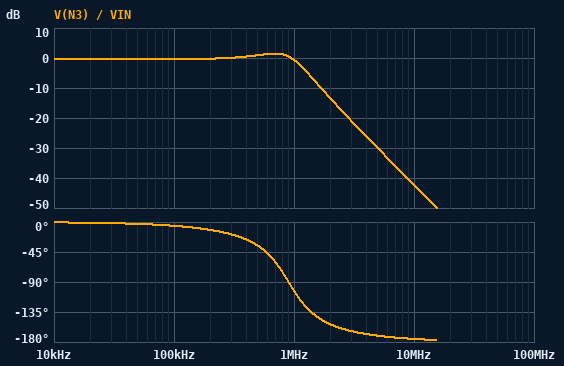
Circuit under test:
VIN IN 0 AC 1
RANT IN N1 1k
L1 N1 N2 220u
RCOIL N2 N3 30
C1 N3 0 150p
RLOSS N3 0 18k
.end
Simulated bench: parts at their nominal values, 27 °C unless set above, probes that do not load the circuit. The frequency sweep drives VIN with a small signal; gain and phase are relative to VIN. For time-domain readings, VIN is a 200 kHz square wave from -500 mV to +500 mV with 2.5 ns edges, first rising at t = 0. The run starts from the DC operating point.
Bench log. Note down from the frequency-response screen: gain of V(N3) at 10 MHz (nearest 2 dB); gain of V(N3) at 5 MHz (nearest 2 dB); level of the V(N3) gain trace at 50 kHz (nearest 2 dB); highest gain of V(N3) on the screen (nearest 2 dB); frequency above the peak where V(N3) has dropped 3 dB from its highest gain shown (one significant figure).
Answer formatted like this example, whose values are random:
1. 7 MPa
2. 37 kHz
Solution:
1. -42 dB
2. -30 dB
3. 0 dB
4. 2 dB
5. 1 MHz
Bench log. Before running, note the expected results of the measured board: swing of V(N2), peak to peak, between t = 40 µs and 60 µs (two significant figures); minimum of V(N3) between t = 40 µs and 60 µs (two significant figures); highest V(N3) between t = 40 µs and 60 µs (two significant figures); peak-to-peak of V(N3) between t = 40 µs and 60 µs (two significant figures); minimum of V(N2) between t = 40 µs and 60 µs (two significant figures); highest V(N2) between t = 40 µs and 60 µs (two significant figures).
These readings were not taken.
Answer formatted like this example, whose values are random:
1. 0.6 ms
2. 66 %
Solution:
1. 1.3 V
2. -670 mV
3. 670 mV
4. 1.3 V
5. -670 mV
6. 670 mV
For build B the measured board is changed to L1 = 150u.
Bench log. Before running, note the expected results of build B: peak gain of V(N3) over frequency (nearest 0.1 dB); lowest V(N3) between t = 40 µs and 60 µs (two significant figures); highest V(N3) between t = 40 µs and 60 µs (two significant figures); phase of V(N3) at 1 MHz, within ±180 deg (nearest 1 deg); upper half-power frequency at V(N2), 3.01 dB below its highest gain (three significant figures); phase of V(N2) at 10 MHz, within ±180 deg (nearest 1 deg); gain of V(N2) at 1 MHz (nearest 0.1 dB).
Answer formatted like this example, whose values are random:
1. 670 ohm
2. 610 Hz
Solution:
1. 0.5 dB
2. -610 mV
3. 610 mV
4. -81 deg
5. 1.26 MHz
6. -158 deg
7. -0.3 dB
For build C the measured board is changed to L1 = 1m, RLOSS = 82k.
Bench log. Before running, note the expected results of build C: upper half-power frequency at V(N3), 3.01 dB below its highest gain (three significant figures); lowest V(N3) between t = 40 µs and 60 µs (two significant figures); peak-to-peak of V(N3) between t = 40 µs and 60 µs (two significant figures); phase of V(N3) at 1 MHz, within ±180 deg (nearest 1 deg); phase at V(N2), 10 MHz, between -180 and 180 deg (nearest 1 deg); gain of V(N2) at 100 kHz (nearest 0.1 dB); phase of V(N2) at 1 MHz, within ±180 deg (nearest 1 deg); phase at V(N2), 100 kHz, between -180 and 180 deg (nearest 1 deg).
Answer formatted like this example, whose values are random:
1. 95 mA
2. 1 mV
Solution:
1. 476 kHz
2. -890 mV
3. 1.8 V
4. -168 deg
5. -163 deg
6. 0.4 dB
7. -166 deg
8. -6 deg
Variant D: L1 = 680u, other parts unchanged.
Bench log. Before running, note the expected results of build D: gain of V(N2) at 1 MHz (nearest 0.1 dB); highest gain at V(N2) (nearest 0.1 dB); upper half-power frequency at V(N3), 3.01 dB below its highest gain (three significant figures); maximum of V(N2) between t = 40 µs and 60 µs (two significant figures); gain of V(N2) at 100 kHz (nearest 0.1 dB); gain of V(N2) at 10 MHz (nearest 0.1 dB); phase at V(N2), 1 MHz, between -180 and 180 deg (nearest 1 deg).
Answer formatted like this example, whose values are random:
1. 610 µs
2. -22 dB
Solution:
1. -10.1 dB
2. 4.6 dB
3. 604 kHz
4. 820 mV
5. -0.2 dB
6. -51.7 dB
7. -156 deg
